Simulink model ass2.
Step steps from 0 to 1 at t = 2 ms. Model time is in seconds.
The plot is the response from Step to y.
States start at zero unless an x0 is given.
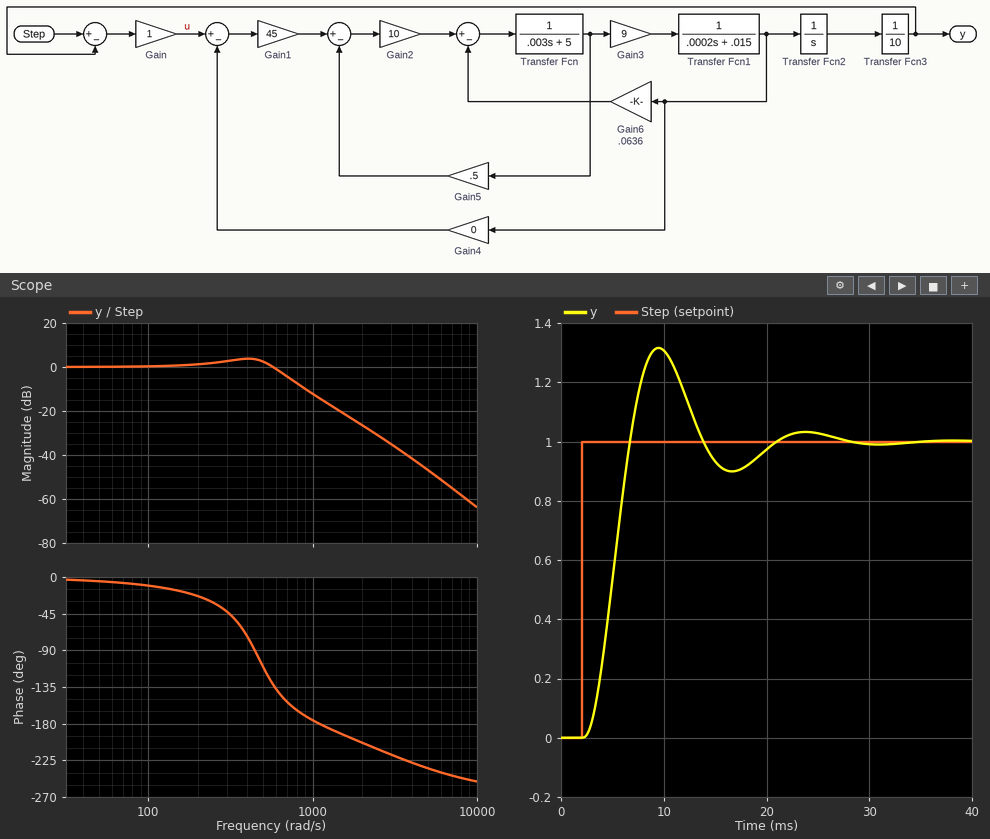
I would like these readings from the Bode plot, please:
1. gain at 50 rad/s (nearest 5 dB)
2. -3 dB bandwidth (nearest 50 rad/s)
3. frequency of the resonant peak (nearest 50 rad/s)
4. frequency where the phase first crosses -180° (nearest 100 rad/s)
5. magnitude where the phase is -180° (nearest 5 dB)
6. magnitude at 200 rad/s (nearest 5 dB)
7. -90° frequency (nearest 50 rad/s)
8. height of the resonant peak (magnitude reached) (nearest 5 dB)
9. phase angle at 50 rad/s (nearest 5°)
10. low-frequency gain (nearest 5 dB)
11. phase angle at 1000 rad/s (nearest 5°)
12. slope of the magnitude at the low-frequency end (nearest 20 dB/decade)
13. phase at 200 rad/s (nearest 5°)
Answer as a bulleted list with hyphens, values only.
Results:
- 0 dB
- 650 rad/s
- 400 rad/s
- 1100 rad/s
- -15 dB
- 0 dB
- 450 rad/s
- 5 dB
- -5°
- 0 dB
- -175°
- 0 dB/decade
- -25°
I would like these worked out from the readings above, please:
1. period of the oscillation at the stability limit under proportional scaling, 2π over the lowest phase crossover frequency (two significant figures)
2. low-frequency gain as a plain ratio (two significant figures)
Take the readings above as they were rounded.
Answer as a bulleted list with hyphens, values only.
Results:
- 0.0057 s
- 1.0
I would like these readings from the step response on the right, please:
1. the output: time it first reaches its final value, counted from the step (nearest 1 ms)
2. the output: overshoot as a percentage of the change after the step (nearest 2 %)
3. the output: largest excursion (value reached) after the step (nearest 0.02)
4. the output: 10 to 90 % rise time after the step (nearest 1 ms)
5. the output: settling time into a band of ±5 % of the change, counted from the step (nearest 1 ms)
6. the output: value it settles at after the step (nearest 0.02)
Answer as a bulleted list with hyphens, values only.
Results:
- 5 ms
- 32 %
- 1.32
- 3 ms
- 17 ms
- 1.00
